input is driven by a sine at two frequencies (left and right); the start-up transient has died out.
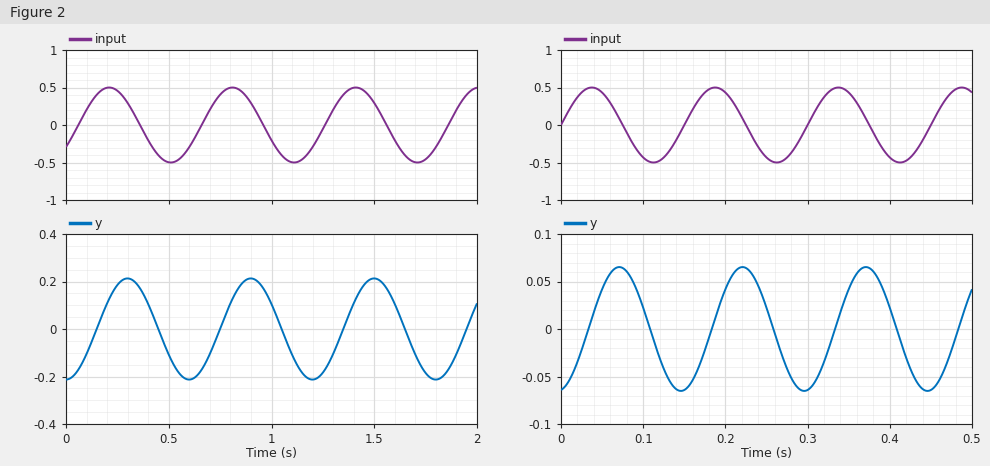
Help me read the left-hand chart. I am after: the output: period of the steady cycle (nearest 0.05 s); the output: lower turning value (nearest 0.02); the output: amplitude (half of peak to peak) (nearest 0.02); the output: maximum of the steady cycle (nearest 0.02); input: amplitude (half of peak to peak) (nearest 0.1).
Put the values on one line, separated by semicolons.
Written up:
0.60 s; -0.22; 0.22; 0.22; 0.5
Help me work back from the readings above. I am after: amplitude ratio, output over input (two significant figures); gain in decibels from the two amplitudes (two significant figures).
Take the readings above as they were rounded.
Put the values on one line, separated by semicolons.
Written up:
0.44; -7.1 dB
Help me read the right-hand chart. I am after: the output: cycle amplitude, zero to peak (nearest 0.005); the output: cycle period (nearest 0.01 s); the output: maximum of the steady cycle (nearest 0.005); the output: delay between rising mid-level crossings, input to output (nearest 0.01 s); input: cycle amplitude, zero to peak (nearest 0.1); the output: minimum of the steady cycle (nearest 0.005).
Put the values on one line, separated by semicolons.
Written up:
0.065; 0.15 s; 0.065; 0.03 s; 0.5; -0.065
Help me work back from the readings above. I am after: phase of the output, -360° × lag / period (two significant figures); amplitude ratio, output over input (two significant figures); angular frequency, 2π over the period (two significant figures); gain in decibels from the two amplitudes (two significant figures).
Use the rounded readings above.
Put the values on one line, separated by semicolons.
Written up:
-72°; 0.13; 42 rad/s; -18 dB
